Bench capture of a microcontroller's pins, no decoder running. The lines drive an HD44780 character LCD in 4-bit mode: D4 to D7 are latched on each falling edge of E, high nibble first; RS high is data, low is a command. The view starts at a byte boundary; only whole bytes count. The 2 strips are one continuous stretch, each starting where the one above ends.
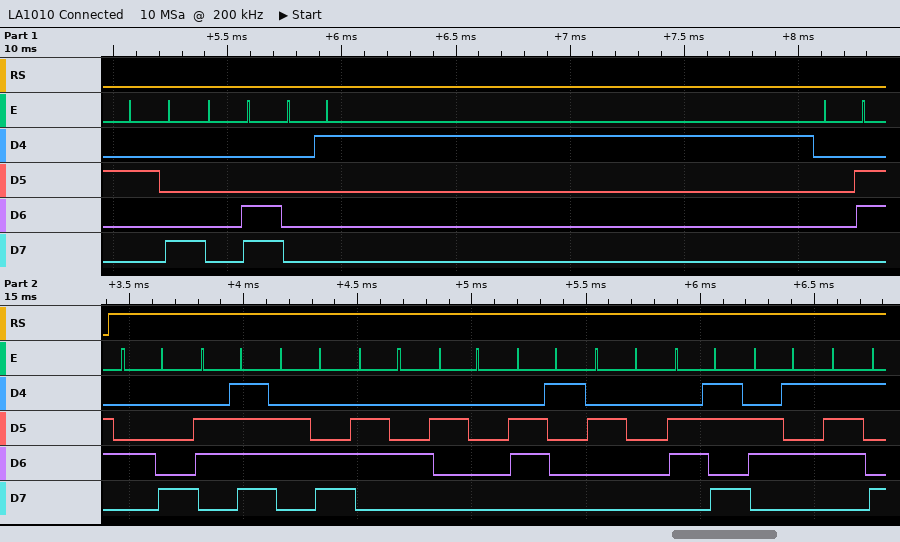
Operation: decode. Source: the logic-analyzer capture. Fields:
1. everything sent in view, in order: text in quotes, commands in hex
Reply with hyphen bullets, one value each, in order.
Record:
- 0x28 0x0C 0x01 0x06 "Hold a key"
